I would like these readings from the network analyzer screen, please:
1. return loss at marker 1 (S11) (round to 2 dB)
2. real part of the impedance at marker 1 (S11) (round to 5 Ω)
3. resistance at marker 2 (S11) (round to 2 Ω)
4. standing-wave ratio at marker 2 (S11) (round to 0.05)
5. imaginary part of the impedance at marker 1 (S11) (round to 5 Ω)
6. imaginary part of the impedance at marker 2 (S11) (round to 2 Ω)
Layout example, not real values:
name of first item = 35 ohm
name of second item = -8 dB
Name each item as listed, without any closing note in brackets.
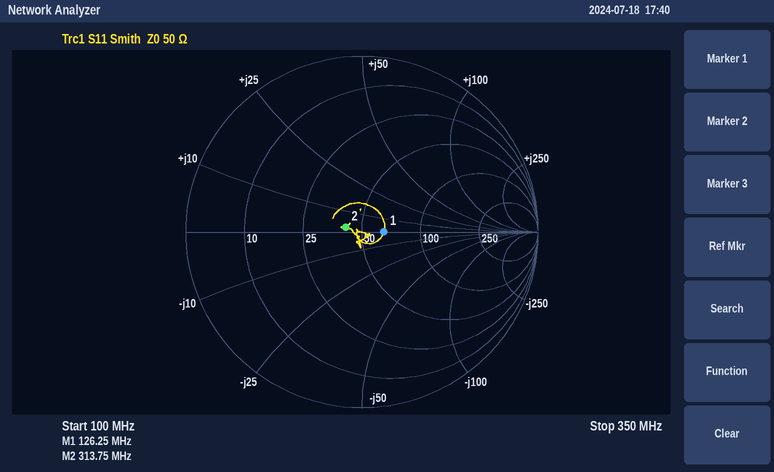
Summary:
return loss at marker 1 (S11) = 18 dB
real part of the impedance at marker 1 (S11) = 65 Ω
resistance at marker 2 (S11) = 42 Ω
standing-wave ratio at marker 2 (S11) = 1.20
imaginary part of the impedance at marker 1 (S11) = 0 Ω
imaginary part of the impedance at marker 2 (S11) = +2 Ω
